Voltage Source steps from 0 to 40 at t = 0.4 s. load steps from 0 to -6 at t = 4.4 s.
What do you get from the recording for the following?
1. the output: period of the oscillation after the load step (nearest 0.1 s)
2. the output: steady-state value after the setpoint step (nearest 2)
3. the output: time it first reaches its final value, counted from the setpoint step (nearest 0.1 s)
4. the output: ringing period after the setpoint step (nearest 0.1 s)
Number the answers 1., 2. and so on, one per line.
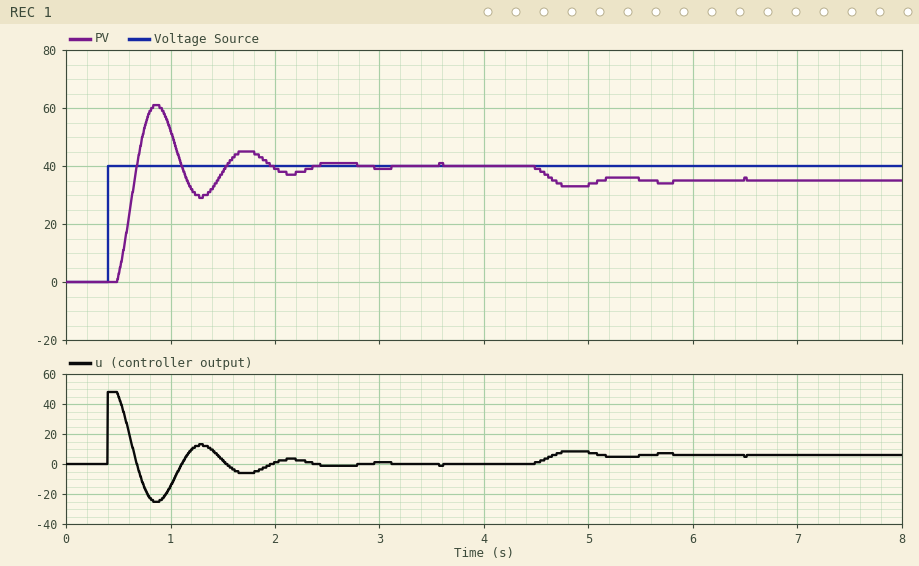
1. 0.9 s
2. 40
3. 0.3 s
4. 0.9 s
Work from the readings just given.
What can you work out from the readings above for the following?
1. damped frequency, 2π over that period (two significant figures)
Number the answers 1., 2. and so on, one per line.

1. 7.0 rad/s
